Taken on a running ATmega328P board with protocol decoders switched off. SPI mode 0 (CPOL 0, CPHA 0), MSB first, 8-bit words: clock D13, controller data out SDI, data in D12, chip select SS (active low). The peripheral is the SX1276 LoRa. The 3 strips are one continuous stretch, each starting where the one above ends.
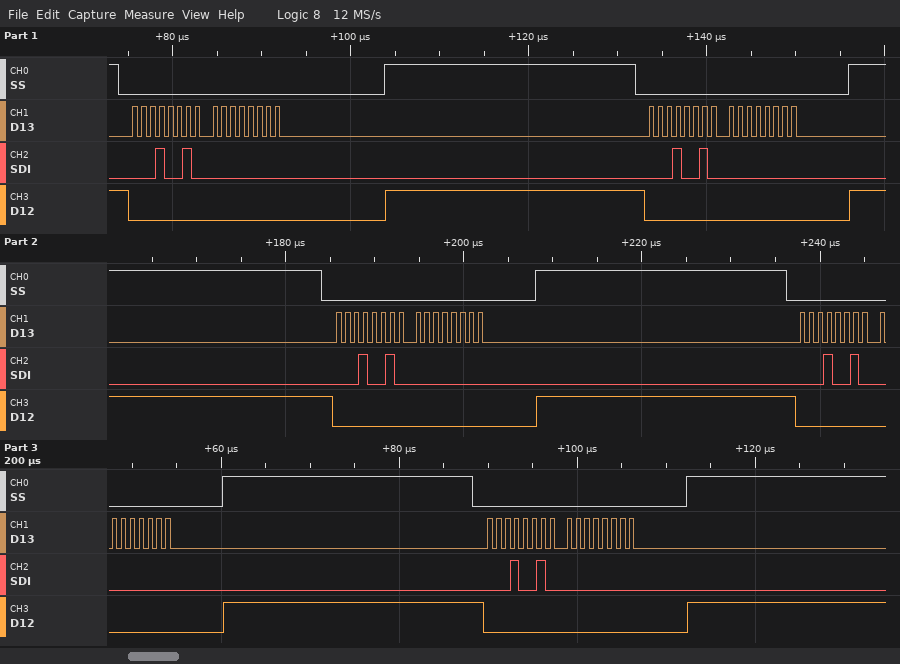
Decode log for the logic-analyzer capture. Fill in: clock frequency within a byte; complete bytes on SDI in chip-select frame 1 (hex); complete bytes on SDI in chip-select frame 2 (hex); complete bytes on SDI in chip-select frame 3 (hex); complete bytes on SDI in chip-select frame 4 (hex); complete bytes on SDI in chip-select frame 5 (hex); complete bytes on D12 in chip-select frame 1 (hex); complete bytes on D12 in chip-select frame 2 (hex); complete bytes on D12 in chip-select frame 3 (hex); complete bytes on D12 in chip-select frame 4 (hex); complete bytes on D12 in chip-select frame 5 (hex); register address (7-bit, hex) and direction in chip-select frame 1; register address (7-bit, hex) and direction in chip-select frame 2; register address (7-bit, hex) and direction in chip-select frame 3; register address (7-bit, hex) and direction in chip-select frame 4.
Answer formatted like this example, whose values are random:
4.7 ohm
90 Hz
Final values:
1 MHz
0x12 0x00
0x12 0x00
0x12 0x00
0x12 0x00
0x12 0x00
0x00 0x00
0x00 0x00
0x00 0x00
0x00 0x00
0x00 0x00
0x12 read
0x12 read
0x12 read
0x12 read
